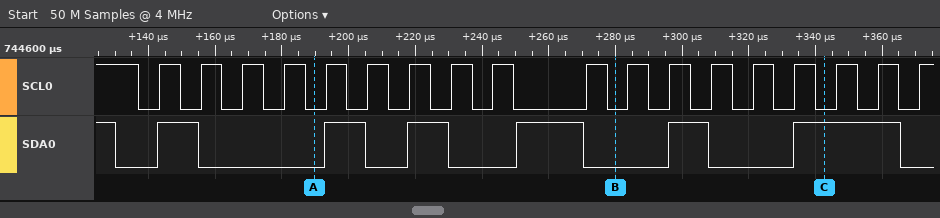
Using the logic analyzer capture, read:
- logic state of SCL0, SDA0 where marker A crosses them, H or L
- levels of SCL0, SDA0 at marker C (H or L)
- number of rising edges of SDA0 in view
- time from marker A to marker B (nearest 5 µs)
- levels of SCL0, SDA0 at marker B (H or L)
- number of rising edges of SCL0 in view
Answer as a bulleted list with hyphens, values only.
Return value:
- SCL0=L, SDA0=L
- SCL0=L, SDA0=H
- 6
- 90 µs
- SCL0=L, SDA0=L
- 18
